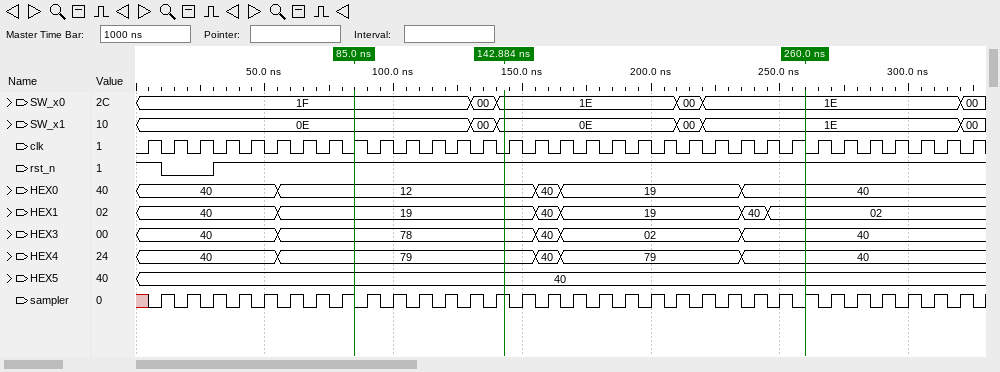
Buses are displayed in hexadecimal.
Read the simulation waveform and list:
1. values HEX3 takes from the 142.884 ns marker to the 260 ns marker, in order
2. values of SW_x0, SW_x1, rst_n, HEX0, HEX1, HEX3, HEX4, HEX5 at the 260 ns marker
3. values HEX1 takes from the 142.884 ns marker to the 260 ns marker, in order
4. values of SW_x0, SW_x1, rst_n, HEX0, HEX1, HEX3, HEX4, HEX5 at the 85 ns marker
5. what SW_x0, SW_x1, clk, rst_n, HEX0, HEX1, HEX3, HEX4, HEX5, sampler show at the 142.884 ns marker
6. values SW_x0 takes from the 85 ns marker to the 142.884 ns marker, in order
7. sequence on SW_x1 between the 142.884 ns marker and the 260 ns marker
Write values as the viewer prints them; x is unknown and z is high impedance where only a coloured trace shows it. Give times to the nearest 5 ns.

78, 40, 02, 40
SW_x0=1E, SW_x1=1E, rst_n=1, HEX0=40, HEX1=02, HEX3=40, HEX4=40, HEX5=40
19, 40, 19, 40, 02
SW_x0=1F, SW_x1=0E, rst_n=1, HEX0=12, HEX1=19, HEX3=78, HEX4=79, HEX5=40
SW_x0=1E, SW_x1=0E, clk=0, rst_n=1, HEX0=12, HEX1=19, HEX3=78, HEX4=79, HEX5=40, sampler=1
1F, 00, 1E
0E, 00, 1E
